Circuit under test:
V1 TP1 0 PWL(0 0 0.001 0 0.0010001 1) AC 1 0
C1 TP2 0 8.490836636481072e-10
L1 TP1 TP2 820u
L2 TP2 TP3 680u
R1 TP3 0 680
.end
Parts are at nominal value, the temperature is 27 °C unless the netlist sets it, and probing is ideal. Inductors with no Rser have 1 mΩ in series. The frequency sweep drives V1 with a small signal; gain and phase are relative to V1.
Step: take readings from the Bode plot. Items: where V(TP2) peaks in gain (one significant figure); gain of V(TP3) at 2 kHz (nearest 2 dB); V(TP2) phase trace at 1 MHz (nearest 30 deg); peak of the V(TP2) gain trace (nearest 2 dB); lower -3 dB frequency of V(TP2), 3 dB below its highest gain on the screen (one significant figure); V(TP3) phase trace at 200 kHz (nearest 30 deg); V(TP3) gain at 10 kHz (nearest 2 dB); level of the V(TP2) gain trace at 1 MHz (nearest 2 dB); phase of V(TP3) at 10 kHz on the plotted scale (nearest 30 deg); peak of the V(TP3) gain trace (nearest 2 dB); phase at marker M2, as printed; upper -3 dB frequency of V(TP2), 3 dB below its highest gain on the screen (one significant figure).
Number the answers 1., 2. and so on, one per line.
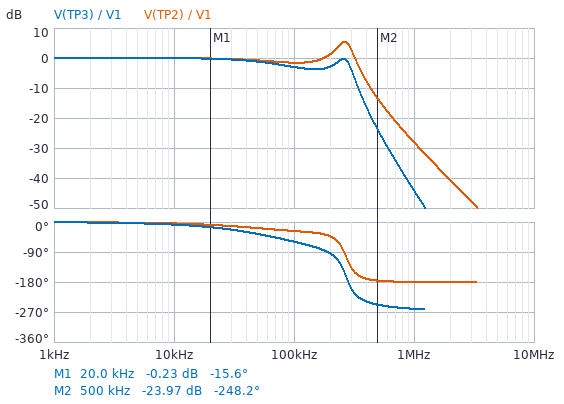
1. 300 kHz
2. 0 dB
3. -180 deg
4. 6 dB
5. 200 kHz
6. -90 deg
7. 0 dB
8. -28 dB
9. 0 deg
10. 0 dB
11. -248.2 deg
12. 300 kHz
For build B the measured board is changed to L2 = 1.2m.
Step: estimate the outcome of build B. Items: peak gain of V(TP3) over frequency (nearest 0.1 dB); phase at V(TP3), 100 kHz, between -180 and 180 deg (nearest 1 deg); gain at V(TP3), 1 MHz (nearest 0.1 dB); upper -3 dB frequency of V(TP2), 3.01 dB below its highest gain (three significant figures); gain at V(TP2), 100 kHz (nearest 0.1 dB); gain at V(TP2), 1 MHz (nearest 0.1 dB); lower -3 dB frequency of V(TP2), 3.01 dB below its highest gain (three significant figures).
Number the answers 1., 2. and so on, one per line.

1. 3.9 dB
2. -65 deg
3. -49.2 dB
4. 259 kHz
5. -1.2 dB
6. -28.2 dB
7. 224 kHz
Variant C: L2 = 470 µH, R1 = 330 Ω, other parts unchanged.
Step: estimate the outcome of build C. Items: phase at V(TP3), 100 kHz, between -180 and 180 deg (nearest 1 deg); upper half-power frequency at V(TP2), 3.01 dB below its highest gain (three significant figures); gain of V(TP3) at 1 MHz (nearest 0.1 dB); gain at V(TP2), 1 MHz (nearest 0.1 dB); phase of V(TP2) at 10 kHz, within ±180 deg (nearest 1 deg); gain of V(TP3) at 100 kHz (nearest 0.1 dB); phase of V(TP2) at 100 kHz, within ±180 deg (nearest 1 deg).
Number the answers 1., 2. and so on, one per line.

1. -72 deg
2. 340 kHz
3. -47.0 dB
4. -27.9 dB
5. -9 deg
6. -7.3 dB
7. -30 deg
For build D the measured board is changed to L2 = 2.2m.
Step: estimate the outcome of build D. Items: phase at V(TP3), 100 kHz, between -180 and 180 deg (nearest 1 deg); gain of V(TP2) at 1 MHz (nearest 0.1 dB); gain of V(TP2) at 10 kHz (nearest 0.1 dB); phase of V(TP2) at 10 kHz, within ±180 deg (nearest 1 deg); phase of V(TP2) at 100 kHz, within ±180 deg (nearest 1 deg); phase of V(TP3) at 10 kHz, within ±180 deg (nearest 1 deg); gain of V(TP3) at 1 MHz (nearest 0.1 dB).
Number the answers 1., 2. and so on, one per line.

1. -72 deg
2. -28.3 dB
3. -0.1 dB
4. -4 deg
5. -8 deg
6. -16 deg
7. -54.5 dB
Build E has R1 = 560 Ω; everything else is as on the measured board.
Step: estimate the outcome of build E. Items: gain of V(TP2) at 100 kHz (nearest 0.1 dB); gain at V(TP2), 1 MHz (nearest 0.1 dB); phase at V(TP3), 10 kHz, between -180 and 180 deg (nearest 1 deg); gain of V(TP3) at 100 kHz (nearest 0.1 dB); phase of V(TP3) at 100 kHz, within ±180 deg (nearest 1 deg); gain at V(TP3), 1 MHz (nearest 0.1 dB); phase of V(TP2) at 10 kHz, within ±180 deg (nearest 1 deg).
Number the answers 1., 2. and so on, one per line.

1. -2.3 dB
2. -28.1 dB
3. -10 deg
4. -4.3 dB
5. -64 deg
6. -45.8 dB
7. -5 deg
